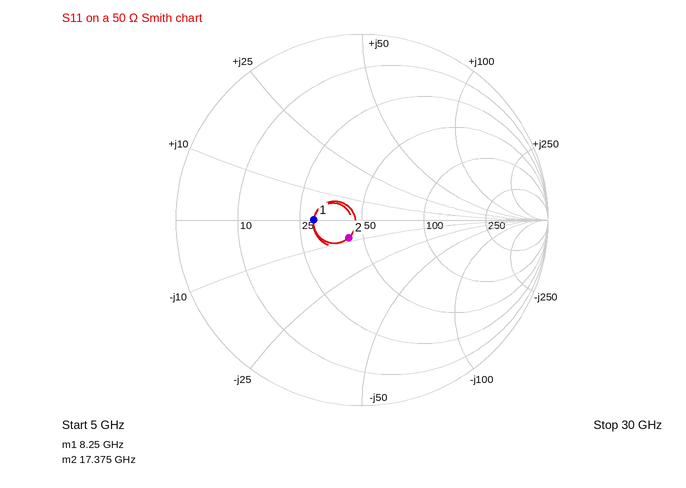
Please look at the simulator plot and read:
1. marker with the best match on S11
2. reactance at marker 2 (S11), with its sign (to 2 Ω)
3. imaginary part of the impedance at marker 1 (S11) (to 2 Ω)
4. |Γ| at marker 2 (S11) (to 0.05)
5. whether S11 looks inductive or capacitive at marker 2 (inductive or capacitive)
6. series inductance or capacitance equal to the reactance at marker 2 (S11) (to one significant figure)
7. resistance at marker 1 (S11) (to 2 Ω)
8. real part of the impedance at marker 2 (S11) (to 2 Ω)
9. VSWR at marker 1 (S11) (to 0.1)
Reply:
marker 2
-8 Ω
0 Ω
0.10
capacitive
1 pF
30 Ω
42 Ω
1.7
